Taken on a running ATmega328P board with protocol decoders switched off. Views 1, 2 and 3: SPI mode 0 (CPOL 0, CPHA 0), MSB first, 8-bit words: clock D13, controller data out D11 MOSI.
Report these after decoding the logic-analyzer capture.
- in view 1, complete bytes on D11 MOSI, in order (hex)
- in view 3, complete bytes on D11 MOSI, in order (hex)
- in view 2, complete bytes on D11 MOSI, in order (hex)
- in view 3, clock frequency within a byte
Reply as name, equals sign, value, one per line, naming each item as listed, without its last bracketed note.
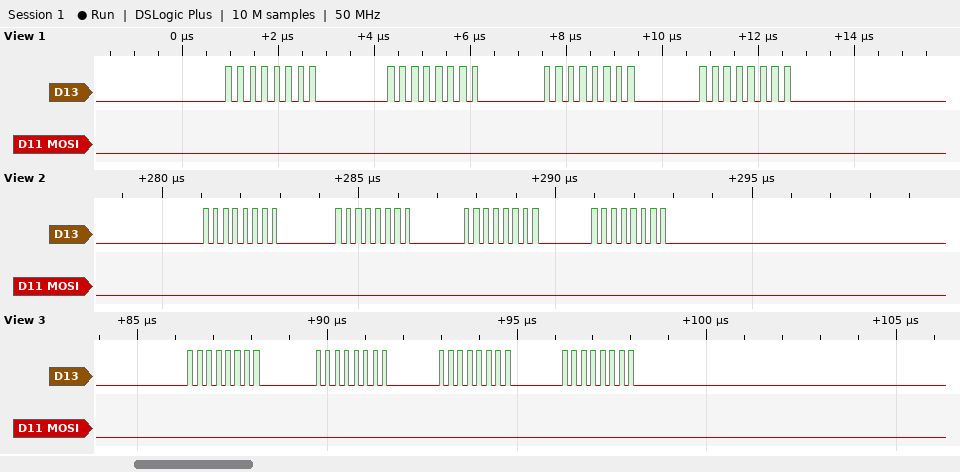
in view 1, complete bytes on D11 MOSI, in order = 00 00 00 00
in view 3, complete bytes on D11 MOSI, in order = 00 00 00 00
in view 2, complete bytes on D11 MOSI, in order = 00 00 00 00
in view 3, clock frequency within a byte = 4 MHz
